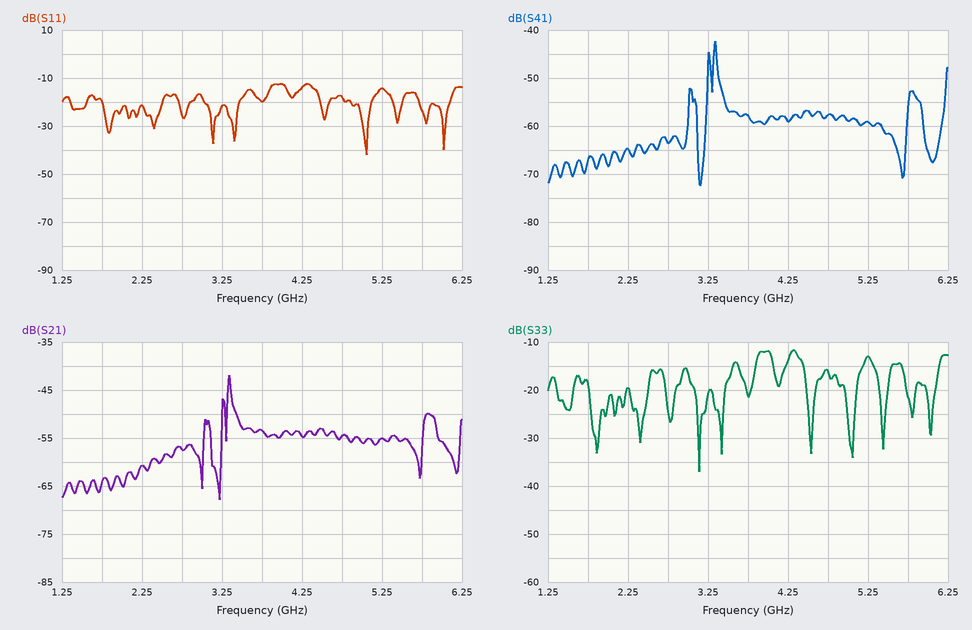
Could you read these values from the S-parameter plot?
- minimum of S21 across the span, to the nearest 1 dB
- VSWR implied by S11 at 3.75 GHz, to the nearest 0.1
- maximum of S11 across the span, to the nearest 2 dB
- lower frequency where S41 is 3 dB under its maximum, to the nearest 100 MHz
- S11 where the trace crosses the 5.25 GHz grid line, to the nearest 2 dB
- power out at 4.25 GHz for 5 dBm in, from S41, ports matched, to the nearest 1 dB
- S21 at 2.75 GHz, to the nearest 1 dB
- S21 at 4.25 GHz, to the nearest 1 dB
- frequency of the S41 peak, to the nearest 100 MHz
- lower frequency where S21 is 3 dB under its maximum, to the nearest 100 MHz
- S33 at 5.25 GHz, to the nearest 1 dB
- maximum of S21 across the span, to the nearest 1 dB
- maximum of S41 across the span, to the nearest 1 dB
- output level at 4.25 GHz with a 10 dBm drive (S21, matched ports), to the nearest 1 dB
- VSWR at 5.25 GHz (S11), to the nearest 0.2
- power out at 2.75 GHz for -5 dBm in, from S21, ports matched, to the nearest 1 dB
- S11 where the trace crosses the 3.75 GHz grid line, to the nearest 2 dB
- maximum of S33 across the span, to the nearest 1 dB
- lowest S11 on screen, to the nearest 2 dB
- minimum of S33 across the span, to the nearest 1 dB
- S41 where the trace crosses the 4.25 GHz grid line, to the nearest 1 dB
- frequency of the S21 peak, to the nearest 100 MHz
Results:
-68 dB
1.2
-12 dB
3.3 GHz
-14 dB
-54 dBm
-57 dB
-55 dB
3.3 GHz
3.3 GHz
-13 dB
-42 dB
-42 dB
-45 dBm
1.4
-62 dBm
-20 dB
-12 dB
-42 dB
-37 dB
-59 dB
3.3 GHz
